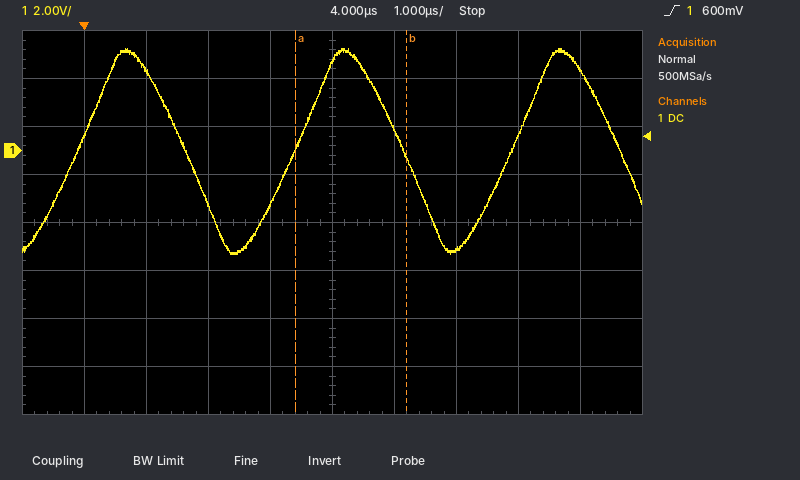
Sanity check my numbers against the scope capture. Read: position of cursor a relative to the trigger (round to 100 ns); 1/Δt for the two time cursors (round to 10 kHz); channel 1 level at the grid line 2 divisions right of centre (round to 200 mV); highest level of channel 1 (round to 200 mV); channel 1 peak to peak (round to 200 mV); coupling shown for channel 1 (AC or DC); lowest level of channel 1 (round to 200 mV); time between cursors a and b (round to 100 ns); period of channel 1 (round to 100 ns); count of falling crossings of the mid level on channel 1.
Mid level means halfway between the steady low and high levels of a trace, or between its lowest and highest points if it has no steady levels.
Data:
+3.4 µs
560 kHz
-4.2 V
4.2 V
8.6 V
DC
-4.4 V
1.8 µs
3.5 µs
3
